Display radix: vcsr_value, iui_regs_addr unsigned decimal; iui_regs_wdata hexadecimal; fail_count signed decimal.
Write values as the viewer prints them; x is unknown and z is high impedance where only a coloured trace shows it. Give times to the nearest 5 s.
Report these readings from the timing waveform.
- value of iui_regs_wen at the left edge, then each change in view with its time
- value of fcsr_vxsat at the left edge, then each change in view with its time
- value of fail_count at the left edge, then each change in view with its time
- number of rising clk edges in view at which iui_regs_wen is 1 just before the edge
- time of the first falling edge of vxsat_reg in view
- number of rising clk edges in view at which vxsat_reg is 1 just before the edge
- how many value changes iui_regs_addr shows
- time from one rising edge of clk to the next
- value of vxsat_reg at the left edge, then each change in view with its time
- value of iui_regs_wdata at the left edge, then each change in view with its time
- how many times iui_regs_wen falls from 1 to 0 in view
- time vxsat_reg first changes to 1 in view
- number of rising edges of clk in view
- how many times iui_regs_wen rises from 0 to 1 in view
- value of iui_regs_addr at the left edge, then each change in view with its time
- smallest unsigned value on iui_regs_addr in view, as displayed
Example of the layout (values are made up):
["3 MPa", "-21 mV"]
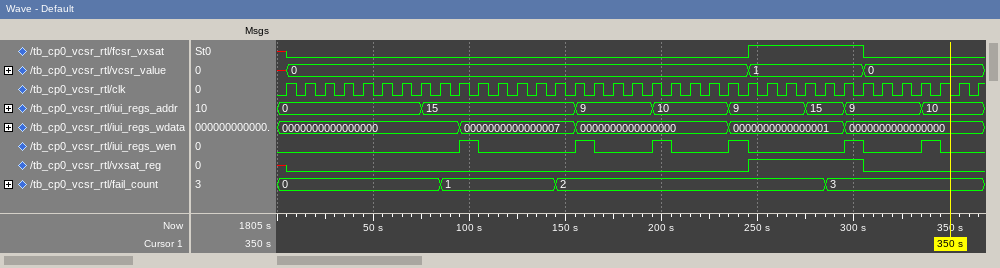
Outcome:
["0, 1 at 95 s, 0 at 105 s, 1 at 155 s, 0 at 165 s, 1 at 195 s, 0 at 205 s, 1 at 235 s, 0 at 245 s, 1 at 295 s, 0 at 305 s, 1 at 335 s, 0 at 345 s", "x, 0 at 5 s, 1 at 245 s, 0 at 305 s", "0, 1 at 85 s, 2 at 145 s, 3 at 285 s", "6", "305 s", "6", "7", "10 s", "x, 0 at 5 s, 1 at 245 s, 0 at 305 s", "0000000000000000, 0000000000000007 at 95 s, 0000000000000000 at 155 s, 0000000000000001 at 235 s, 0000000000000000 at 295 s", "6", "245 s", "37", "6", "0, 15 at 75 s, 9 at 155 s, 10 at 195 s, 9 at 235 s, 15 at 275 s, 9 at 295 s, 10 at 335 s", "0"]
